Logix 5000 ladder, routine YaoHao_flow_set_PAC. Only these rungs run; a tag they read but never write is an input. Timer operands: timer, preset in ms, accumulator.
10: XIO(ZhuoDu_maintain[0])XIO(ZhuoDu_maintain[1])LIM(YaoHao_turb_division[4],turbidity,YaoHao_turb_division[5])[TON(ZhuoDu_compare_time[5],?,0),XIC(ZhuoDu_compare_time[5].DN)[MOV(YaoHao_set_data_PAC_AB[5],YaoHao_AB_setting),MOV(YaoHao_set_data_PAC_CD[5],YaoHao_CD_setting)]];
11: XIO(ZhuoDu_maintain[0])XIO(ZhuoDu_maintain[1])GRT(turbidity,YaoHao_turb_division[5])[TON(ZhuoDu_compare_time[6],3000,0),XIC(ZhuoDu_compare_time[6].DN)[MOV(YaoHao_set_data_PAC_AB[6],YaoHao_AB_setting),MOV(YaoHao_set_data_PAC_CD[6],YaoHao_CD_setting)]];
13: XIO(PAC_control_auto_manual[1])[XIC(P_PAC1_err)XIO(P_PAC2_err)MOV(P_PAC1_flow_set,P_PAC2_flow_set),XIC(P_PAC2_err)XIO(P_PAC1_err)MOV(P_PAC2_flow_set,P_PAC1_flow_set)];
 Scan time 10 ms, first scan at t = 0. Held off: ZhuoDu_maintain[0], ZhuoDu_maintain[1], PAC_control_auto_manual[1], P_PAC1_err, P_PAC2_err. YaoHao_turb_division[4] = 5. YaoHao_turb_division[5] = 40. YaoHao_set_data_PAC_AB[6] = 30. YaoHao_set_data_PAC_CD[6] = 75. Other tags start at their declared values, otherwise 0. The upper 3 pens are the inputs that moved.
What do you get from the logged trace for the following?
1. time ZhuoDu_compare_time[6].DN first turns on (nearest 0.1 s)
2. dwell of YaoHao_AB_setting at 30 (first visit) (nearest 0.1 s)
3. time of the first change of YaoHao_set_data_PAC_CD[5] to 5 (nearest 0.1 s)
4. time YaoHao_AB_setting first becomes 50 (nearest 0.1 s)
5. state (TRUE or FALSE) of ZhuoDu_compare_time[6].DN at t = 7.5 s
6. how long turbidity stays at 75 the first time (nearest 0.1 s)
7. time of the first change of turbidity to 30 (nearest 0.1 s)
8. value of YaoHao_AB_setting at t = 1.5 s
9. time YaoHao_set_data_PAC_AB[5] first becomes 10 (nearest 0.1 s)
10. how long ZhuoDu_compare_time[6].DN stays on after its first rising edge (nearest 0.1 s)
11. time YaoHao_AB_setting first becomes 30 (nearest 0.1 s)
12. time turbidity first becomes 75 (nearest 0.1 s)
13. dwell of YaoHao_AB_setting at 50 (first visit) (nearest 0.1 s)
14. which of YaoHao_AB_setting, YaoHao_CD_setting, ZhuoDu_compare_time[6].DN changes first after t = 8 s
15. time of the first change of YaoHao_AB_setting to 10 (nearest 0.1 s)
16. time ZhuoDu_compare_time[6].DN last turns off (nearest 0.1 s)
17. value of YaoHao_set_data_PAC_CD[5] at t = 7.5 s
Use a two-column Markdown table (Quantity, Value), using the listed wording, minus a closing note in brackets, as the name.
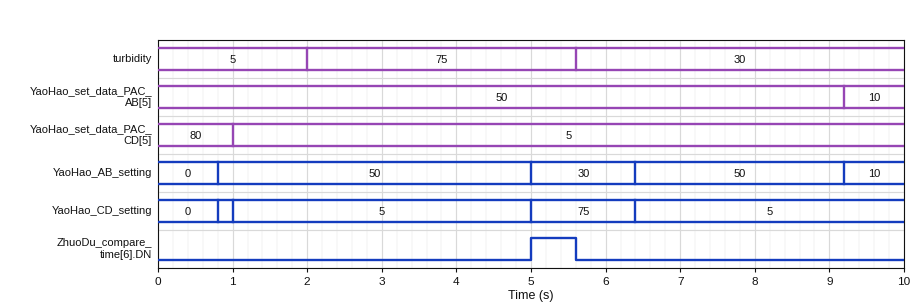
| Quantity | Value |
|---|---|
| time ZhuoDu_compare_time[6].DN first turns on | 5.0 s |
| dwell of YaoHao_AB_setting at 30 (first visit) | 1.4 s |
| time of the first change of YaoHao_set_data_PAC_CD[5] to 5 | 1.0 s |
| time YaoHao_AB_setting first becomes 50 | 0.8 s |
| state (TRUE or FALSE) of ZhuoDu_compare_time[6].DN at t = 7.5 s | FALSE |
| how long turbidity stays at 75 the first time | 3.6 s |
| time of the first change of turbidity to 30 | 5.6 s |
| value of YaoHao_AB_setting at t = 1.5 s | 50 |
| time YaoHao_set_data_PAC_AB[5] first becomes 10 | 9.2 s |
| how long ZhuoDu_compare_time[6].DN stays on after its first rising edge | 0.6 s |
| time YaoHao_AB_setting first becomes 30 | 5.0 s |
| time turbidity first becomes 75 | 2.0 s |
| dwell of YaoHao_AB_setting at 50 (first visit) | 4.2 s |
| which of YaoHao_AB_setting, YaoHao_CD_setting, ZhuoDu_compare_time[6].DN changes first after t = 8 s | YaoHao_AB_setting |
| time of the first change of YaoHao_AB_setting to 10 | 9.2 s |
| time ZhuoDu_compare_time[6].DN last turns off | 5.6 s |
| value of YaoHao_set_data_PAC_CD[5] at t = 7.5 s | 5 |
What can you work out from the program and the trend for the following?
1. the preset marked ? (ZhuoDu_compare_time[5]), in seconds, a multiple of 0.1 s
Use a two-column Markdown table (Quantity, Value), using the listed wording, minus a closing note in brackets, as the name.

| Quantity | Value |
|---|---|
| the preset marked ? (ZhuoDu_compare_time[5]), in seconds, a multiple of 0.1 s | 0.8 s |
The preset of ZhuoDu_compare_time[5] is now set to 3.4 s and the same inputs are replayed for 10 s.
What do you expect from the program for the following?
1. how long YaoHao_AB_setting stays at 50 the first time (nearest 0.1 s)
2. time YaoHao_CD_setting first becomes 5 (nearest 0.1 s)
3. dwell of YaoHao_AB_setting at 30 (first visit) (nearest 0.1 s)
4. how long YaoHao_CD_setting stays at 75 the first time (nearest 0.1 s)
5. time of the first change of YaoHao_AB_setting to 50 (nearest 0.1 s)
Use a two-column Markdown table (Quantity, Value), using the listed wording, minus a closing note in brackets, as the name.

| Quantity | Value |
|---|---|
| how long YaoHao_AB_setting stays at 50 the first time | 0.2 s |
| time YaoHao_CD_setting first becomes 5 | 9.0 s |
| dwell of YaoHao_AB_setting at 30 (first visit) | 4.0 s |
| how long YaoHao_CD_setting stays at 75 the first time | 4.0 s |
| time of the first change of YaoHao_AB_setting to 50 | 9.0 s |
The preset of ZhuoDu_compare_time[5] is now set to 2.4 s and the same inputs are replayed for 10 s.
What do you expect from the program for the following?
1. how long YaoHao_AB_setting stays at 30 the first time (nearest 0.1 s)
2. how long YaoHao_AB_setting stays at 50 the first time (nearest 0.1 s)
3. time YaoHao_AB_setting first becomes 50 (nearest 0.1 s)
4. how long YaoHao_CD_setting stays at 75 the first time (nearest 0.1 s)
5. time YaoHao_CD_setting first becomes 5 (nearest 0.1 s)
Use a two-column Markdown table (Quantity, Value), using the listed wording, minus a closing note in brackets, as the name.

| Quantity | Value |
|---|---|
| how long YaoHao_AB_setting stays at 30 the first time | 3.0 s |
| how long YaoHao_AB_setting stays at 50 the first time | 1.2 s |
| time YaoHao_AB_setting first becomes 50 | 8.0 s |
| how long YaoHao_CD_setting stays at 75 the first time | 3.0 s |
| time YaoHao_CD_setting first becomes 5 | 8.0 s |
